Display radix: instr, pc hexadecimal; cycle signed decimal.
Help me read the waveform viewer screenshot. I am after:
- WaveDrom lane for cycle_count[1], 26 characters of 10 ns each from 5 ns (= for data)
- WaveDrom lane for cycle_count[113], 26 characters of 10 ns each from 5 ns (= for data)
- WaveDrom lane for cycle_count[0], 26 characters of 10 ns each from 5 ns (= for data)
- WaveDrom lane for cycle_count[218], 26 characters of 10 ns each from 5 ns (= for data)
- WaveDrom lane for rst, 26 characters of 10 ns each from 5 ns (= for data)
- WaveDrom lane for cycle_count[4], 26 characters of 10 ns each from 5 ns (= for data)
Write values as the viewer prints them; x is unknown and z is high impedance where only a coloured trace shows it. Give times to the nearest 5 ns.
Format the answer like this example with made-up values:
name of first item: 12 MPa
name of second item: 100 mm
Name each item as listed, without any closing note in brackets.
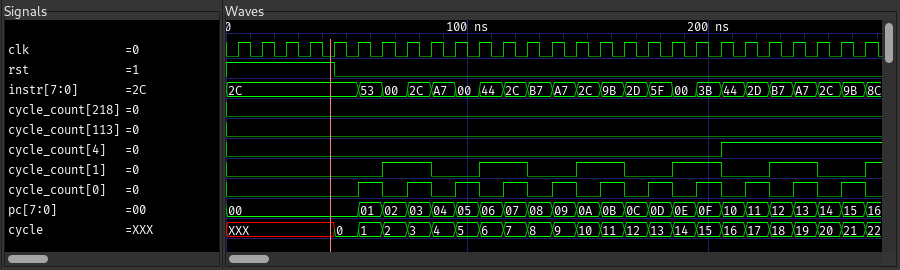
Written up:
WaveDrom lane for cycle_count[1], 26 characters of 10 ns each from 5 ns: {name: 'cycle_count[1]', wave: '0.....1.0.1.0.1.0.1.0.1.0.'}
WaveDrom lane for cycle_count[113], 26 characters of 10 ns each from 5 ns: {name: 'cycle_count[113]', wave: '0.........................'}
WaveDrom lane for cycle_count[0], 26 characters of 10 ns each from 5 ns: {name: 'cycle_count[0]', wave: '0....101010101010101010101'}
WaveDrom lane for cycle_count[218], 26 characters of 10 ns each from 5 ns: {name: 'cycle_count[218]', wave: '0.........................'}
WaveDrom lane for rst, 26 characters of 10 ns each from 5 ns: {name: 'rst', wave: '1...0.....................'}
WaveDrom lane for cycle_count[4], 26 characters of 10 ns each from 5 ns: {name: 'cycle_count[4]', wave: '0...................1.....'}
